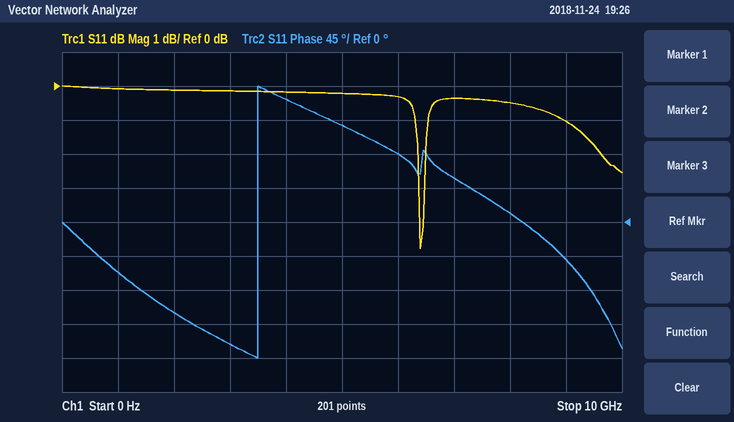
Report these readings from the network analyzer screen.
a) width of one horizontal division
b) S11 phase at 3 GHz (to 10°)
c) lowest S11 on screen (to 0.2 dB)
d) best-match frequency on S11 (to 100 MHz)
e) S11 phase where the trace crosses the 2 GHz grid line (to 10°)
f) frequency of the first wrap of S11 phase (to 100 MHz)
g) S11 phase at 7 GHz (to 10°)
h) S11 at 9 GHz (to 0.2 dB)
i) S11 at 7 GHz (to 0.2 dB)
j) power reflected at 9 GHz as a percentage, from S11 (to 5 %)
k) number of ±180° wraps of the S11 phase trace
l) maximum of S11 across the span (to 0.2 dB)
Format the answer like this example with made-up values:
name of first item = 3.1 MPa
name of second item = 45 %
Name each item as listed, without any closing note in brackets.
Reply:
width of one horizontal division = 1 GHz
S11 phase at 3 GHz = -160°
lowest S11 on screen = -4.8 dB
best-match frequency on S11 = 6.4 GHz
S11 phase where the trace crosses the 2 GHz grid line = -120°
frequency of the first wrap of S11 phase = 3.5 GHz
S11 phase at 7 GHz = 60°
S11 at 9 GHz = -1.0 dB
S11 at 7 GHz = -0.4 dB
power reflected at 9 GHz as a percentage, from S11 = 80 %
number of ±180° wraps of the S11 phase trace = 1
maximum of S11 across the span = 0.0 dB
